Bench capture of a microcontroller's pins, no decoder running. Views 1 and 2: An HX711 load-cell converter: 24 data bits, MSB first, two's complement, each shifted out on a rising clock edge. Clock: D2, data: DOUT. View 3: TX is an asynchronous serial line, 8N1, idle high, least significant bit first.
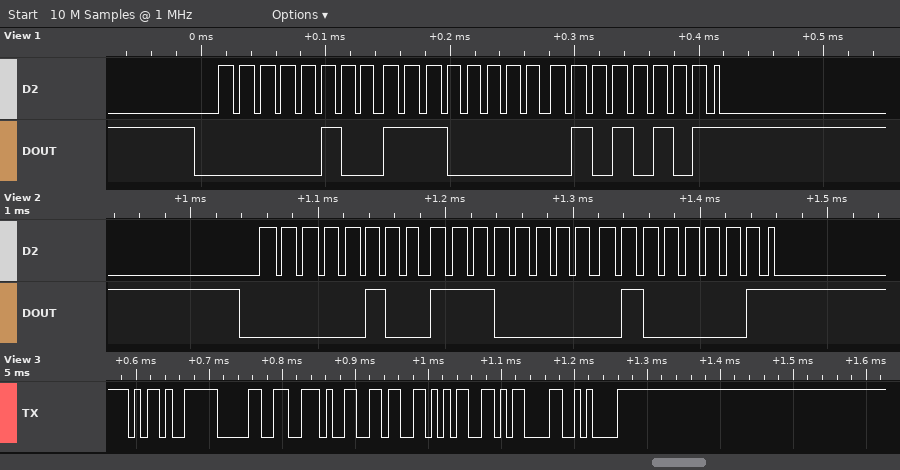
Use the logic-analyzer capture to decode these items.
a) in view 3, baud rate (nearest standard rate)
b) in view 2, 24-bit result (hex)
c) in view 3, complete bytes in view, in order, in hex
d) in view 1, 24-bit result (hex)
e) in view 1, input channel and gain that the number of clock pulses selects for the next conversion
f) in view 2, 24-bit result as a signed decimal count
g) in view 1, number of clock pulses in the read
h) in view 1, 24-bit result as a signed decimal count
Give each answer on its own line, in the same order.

115200 baud
0x04E041
2D 30 2E 36 35 0D 0A
0x04E055
channel A, gain 128
319553
25
319573
